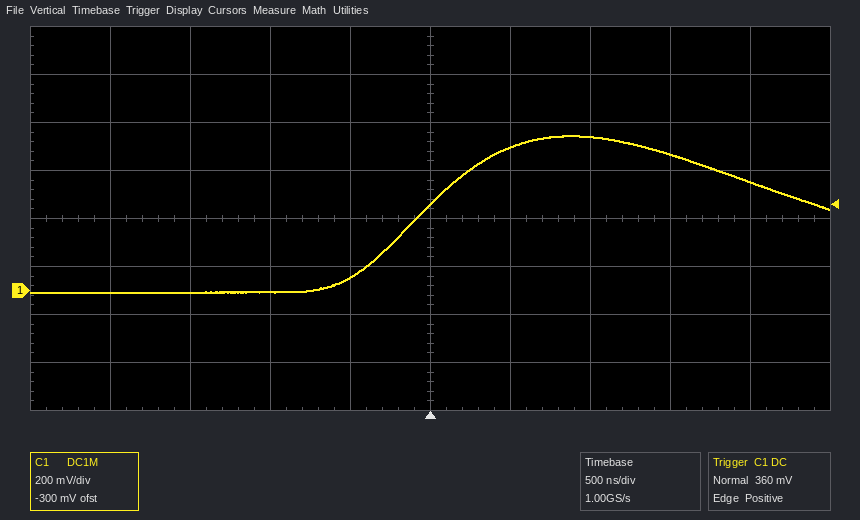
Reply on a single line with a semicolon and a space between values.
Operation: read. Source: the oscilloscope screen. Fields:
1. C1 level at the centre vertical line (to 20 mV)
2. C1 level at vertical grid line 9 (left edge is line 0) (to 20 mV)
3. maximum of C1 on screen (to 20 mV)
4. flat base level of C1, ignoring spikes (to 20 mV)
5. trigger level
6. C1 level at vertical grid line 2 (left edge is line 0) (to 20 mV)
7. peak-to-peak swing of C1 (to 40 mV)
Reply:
360 mV; 460 mV; 640 mV; 0 mV; 360 mV; 0 mV; 640 mV
